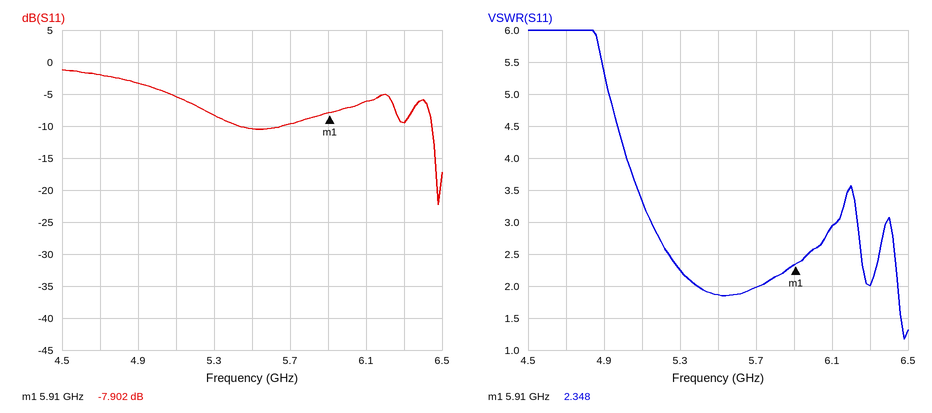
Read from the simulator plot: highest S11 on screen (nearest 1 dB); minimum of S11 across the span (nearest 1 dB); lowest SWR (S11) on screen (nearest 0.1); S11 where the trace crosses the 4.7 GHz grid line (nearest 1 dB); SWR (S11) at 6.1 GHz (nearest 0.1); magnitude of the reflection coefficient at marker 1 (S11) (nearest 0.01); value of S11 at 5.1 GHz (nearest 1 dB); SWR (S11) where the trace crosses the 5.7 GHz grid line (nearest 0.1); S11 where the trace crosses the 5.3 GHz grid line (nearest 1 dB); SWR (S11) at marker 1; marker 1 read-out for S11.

-1 dB
-22 dB
1.2
-2 dB
2.9
0.40
-5 dB
2.0
-8 dB
2.348
-7.902 dB
